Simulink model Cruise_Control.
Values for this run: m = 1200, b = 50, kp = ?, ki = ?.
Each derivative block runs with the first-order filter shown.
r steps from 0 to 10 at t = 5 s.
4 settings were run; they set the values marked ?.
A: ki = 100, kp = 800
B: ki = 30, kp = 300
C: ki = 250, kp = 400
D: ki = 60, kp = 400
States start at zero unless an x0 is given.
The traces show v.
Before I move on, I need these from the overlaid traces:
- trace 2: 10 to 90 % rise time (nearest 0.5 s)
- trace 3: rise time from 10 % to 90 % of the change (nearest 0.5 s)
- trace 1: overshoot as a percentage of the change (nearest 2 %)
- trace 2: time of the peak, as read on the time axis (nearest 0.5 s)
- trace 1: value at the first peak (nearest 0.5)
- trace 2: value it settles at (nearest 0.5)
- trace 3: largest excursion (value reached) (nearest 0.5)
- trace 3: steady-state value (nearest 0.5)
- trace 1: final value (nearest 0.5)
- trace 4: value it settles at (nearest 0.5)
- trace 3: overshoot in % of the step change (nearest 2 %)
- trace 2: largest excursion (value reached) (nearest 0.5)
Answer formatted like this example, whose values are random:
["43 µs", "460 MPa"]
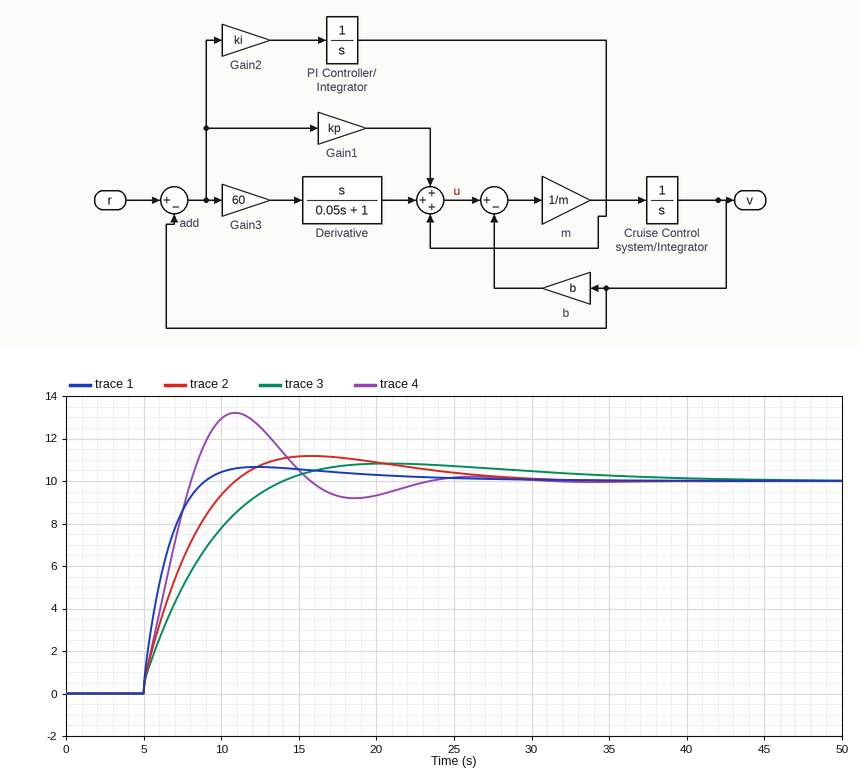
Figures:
["4.5 s", "6.5 s", "6 %", "16.0 s", "10.5", "10.0", "11.0", "10.0", "10.0", "10.0", "8 %", "11.0"]
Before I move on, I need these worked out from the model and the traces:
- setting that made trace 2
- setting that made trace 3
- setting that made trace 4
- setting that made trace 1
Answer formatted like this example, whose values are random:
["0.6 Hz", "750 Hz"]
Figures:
["D", "B", "C", "A"]
